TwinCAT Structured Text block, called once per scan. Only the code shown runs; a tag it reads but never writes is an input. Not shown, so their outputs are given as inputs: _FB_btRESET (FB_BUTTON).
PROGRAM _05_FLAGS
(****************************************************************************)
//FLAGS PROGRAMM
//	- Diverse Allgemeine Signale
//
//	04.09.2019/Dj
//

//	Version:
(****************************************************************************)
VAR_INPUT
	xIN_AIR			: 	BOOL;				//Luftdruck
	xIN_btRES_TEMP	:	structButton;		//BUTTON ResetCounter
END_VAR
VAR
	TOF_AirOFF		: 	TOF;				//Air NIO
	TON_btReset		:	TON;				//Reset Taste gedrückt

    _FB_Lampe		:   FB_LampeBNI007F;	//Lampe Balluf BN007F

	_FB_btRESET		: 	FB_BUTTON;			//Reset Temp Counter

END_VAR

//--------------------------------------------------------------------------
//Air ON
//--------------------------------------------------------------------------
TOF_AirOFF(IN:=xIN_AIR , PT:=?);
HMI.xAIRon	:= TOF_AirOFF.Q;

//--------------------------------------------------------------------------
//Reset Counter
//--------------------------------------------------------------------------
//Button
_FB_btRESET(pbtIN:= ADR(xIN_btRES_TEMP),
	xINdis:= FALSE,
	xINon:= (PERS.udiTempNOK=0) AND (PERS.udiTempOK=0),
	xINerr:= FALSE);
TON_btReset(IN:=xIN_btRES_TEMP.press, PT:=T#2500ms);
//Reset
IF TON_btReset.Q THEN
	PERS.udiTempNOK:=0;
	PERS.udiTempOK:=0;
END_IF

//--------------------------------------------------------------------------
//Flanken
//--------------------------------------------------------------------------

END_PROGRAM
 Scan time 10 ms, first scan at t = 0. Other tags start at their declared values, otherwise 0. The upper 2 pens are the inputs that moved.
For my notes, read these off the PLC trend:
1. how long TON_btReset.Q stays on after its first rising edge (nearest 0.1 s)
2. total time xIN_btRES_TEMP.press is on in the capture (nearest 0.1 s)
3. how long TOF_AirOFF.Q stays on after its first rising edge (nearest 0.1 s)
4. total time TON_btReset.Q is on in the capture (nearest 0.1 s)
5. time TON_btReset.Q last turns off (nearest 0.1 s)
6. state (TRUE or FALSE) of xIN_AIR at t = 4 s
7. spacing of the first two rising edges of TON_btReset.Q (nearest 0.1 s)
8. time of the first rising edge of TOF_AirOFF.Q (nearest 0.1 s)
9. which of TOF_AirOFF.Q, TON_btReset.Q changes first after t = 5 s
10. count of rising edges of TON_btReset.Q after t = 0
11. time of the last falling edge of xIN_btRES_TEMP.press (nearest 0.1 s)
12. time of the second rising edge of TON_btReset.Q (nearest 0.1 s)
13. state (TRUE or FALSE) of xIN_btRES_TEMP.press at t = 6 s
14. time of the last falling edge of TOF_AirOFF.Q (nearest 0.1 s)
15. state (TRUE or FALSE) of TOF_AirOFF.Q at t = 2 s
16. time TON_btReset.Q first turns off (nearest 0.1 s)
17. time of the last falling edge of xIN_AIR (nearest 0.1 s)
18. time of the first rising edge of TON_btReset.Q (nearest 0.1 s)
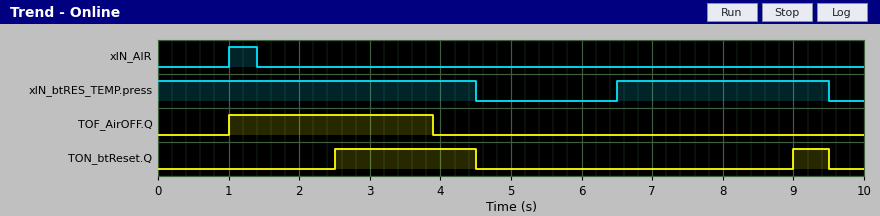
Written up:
2.0 s
7.5 s
2.9 s
2.5 s
9.5 s
FALSE
6.5 s
1.0 s
TON_btReset.Q
2
9.5 s
9.0 s
FALSE
3.9 s
TRUE
4.5 s
1.4 s
2.5 s
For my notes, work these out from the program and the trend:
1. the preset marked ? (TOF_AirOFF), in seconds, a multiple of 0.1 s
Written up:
2.5 s
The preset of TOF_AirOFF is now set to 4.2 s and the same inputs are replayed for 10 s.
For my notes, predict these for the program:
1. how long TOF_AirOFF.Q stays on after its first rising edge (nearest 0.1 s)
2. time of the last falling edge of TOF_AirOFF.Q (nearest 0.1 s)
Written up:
4.6 s
5.6 s
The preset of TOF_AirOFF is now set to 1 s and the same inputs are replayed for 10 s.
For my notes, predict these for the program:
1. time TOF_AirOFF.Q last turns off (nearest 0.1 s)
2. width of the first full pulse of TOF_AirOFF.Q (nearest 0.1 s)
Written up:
2.4 s
1.4 s
